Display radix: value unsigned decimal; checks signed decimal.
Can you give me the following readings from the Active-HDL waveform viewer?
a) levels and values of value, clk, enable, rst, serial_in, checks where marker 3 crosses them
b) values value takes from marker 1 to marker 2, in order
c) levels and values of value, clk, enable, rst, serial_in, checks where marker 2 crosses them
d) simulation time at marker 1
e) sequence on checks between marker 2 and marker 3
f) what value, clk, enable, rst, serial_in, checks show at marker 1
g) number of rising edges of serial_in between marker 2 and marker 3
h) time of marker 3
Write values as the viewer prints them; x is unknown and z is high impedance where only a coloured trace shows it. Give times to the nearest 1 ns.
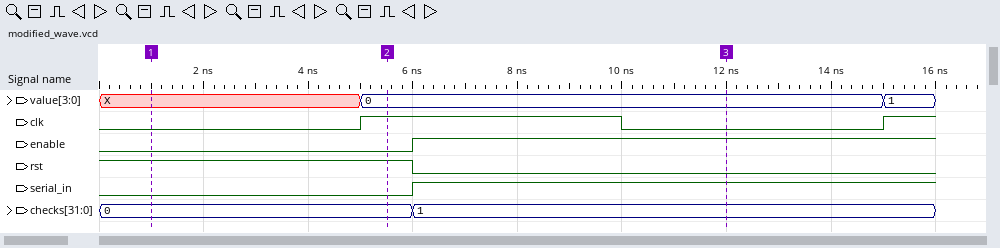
value=0, clk=0, enable=1, rst=0, serial_in=1, checks=1
X, 0
value=0, clk=1, enable=0, rst=1, serial_in=0, checks=0
1 ns
0, 1
value=X, clk=0, enable=0, rst=1, serial_in=0, checks=0
1
12 ns
